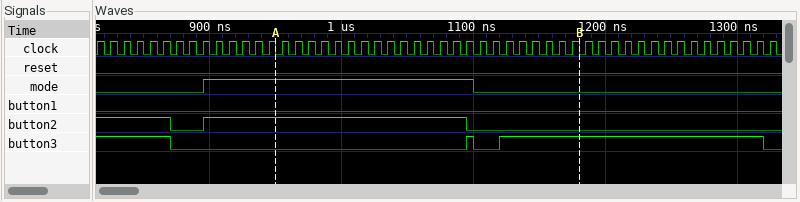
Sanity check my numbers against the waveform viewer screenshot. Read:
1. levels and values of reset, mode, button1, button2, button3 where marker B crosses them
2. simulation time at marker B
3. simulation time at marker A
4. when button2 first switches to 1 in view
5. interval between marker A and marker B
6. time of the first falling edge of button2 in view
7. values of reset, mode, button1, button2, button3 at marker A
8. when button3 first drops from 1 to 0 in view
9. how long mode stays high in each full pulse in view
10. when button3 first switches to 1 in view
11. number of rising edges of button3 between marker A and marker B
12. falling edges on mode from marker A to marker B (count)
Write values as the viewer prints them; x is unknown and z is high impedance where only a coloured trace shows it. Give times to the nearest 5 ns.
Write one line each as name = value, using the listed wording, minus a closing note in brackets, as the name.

levels and values of reset, mode, button1, button2, button3 where marker B crosses them = reset=0, mode=0, button1=0, button2=0, button3=1
simulation time at marker B = 1180 ns
simulation time at marker A = 950 ns
when button2 first switches to 1 in view = 895 ns
interval between marker A and marker B = 230 ns
time of the first falling edge of button2 in view = 870 ns
values of reset, mode, button1, button2, button3 at marker A = reset=0, mode=1, button1=0, button2=1, button3=0
when button3 first drops from 1 to 0 in view = 870 ns
how long mode stays high in each full pulse in view = 205 ns
when button3 first switches to 1 in view = 1095 ns
number of rising edges of button3 between marker A and marker B = 2
falling edges on mode from marker A to marker B = 1
